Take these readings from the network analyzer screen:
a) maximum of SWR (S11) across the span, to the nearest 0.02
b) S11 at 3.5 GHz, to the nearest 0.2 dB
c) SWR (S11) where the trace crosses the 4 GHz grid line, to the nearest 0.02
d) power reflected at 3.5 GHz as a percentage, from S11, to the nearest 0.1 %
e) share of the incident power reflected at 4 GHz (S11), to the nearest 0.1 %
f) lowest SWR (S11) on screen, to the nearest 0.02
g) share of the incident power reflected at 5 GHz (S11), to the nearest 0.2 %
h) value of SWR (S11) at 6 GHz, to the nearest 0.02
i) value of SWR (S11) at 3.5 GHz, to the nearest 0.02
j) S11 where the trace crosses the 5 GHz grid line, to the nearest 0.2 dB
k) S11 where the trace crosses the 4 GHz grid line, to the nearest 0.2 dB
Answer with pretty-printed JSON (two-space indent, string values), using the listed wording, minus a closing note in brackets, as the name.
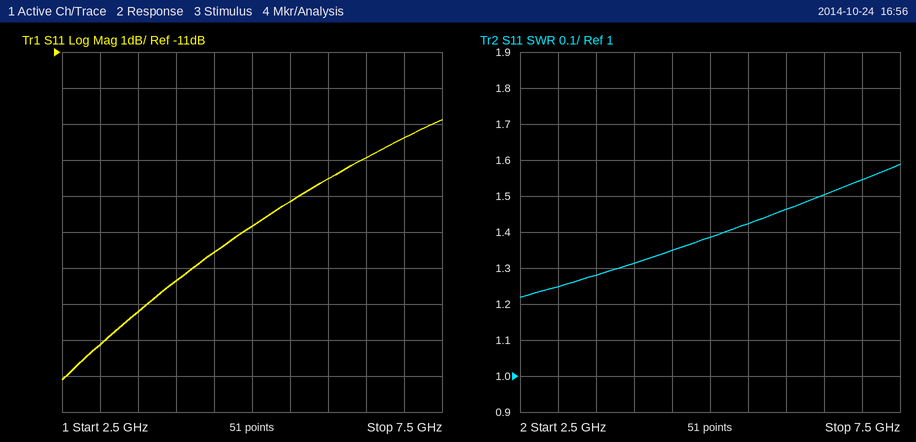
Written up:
{
  "maximum of SWR (S11) across the span, to the nearest 0.02": "1.58",
  "S11 at 3.5 GHz, to the nearest 0.2 dB": "-18.2 dB",
  "SWR (S11) where the trace crosses the 4 GHz grid line, to the nearest 0.02": "1.32",
  "power reflected at 3.5 GHz as a percentage, from S11, to the nearest 0.1 %": "1.5 %",
  "share of the incident power reflected at 4 GHz (S11), to the nearest 0.1 %": "1.8 %",
  "lowest SWR (S11) on screen, to the nearest 0.02": "1.22",
  "share of the incident power reflected at 5 GHz (S11), to the nearest 0.2 %": "2.6 %",
  "value of SWR (S11) at 6 GHz, to the nearest 0.02": "1.46",
  "value of SWR (S11) at 3.5 GHz, to the nearest 0.02": "1.28",
  "S11 where the trace crosses the 5 GHz grid line, to the nearest 0.2 dB": "-15.8 dB",
  "S11 where the trace crosses the 4 GHz grid line, to the nearest 0.2 dB": "-17.4 dB"
}
